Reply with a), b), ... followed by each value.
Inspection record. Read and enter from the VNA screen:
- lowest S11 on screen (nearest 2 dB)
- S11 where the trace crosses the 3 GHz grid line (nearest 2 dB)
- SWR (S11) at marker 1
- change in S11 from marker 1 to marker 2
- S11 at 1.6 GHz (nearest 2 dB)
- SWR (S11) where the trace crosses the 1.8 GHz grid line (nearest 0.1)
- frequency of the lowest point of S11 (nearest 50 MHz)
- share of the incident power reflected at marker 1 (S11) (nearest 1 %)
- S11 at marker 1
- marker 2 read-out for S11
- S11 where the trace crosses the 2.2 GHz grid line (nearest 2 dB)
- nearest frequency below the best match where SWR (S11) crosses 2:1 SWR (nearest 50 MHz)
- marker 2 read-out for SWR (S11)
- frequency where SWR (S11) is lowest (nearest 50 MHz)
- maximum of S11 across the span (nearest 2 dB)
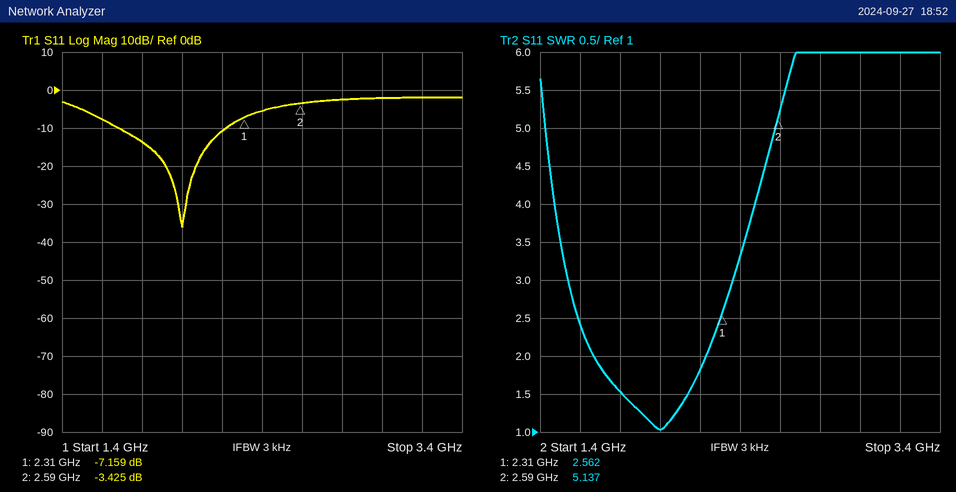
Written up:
a) -36 dB
b) -2 dB
c) 2.562
d) 3.734 dB
e) -8 dB
f) 1.5
g) 2.00 GHz
h) 19 %
i) -7.159 dB
j) -3.425 dB
k) -10 dB
l) 1.65 GHz
m) 5.137
n) 2.00 GHz
o) -2 dB
